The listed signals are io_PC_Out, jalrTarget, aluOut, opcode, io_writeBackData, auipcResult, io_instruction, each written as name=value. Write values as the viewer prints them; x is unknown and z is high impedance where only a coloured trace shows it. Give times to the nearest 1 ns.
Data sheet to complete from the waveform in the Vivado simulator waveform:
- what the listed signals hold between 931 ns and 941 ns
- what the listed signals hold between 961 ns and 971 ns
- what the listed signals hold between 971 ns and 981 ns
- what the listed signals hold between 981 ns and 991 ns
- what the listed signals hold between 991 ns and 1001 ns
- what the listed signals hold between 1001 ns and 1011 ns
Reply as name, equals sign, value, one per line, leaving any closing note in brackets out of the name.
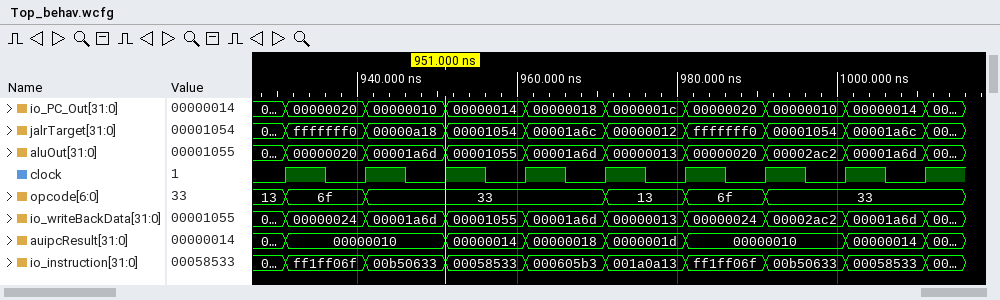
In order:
what the listed signals hold between 931 ns and 941 ns = io_PC_Out=00000020, jalrTarget=fffffff0, aluOut=00000020, opcode=6f, io_writeBackData=00000024, auipcResult=00000010, io_instruction=ff1ff06f
what the listed signals hold between 961 ns and 971 ns = io_PC_Out=00000018, jalrTarget=00001a6c, aluOut=00001a6d, opcode=33, io_writeBackData=00001a6d, auipcResult=00000018, io_instruction=000605b3
what the listed signals hold between 971 ns and 981 ns = io_PC_Out=0000001c, jalrTarget=00000012, aluOut=00000013, opcode=13, io_writeBackData=00000013, auipcResult=0000001d, io_instruction=001a0a13
what the listed signals hold between 981 ns and 991 ns = io_PC_Out=00000020, jalrTarget=fffffff0, aluOut=00000020, opcode=6f, io_writeBackData=00000024, auipcResult=00000010, io_instruction=ff1ff06f
what the listed signals hold between 991 ns and 1001 ns = io_PC_Out=00000010, jalrTarget=00001054, aluOut=00002ac2, opcode=33, io_writeBackData=00002ac2, auipcResult=00000010, io_instruction=00b50633
what the listed signals hold between 1001 ns and 1011 ns = io_PC_Out=00000014, jalrTarget=00001a6c, aluOut=00001a6d, opcode=33, io_writeBackData=00001a6d, auipcResult=00000014, io_instruction=00058533
